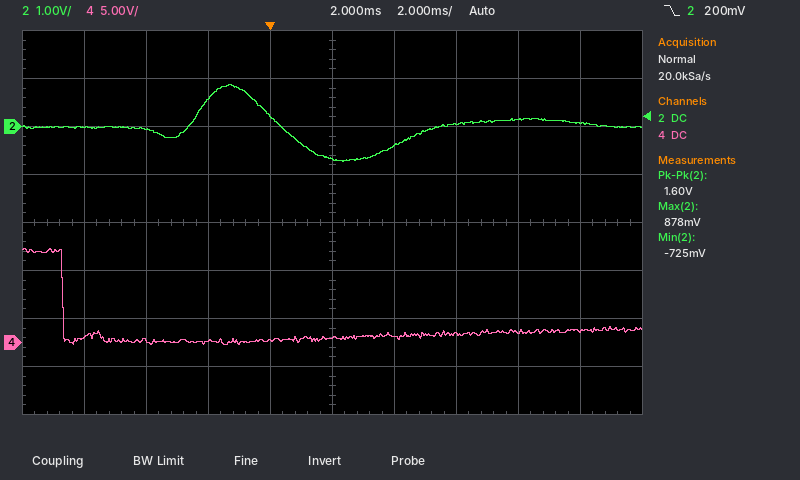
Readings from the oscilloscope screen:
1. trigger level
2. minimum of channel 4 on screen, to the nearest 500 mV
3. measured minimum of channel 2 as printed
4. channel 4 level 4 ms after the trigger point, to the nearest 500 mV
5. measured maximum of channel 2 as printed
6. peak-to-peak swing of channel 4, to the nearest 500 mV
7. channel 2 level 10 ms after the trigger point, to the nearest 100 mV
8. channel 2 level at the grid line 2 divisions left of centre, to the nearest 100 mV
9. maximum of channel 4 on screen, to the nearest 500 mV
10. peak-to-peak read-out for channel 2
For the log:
200 mV
0.0 V
-725 mV
500 mV
878 mV
10.0 V
100 mV
600 mV
10.0 V
1.60 V
